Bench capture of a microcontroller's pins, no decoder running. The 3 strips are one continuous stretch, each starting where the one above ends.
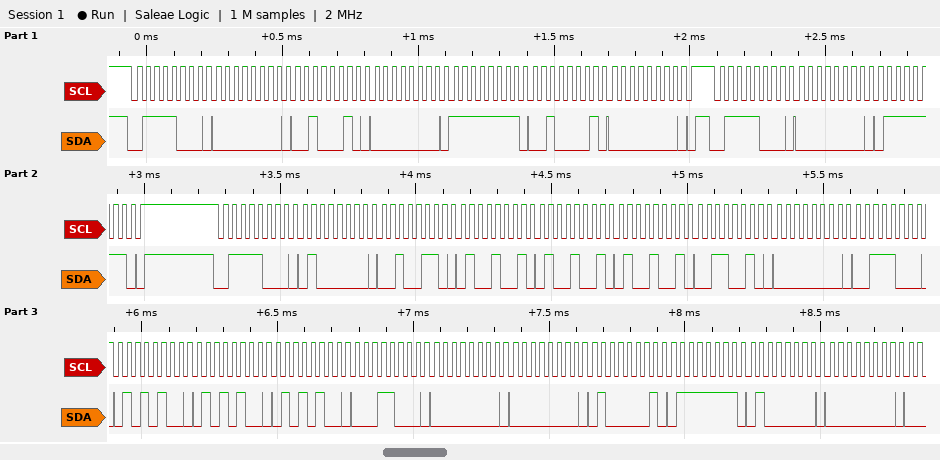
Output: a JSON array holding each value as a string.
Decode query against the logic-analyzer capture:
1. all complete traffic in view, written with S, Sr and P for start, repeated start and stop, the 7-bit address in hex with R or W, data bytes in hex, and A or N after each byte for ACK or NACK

["S 3CW A 00 A 22 A 00 A FF A 21 A 00 A P S 3CW A 00 A 7F A P S 3CW A 40 A 26 A 49 A 49 A 49 A 32 A 00 A 38 A 54 A 54 A 54 A 18 A 00 A 00 A 41 A 7F A 40 A 00 A"]
